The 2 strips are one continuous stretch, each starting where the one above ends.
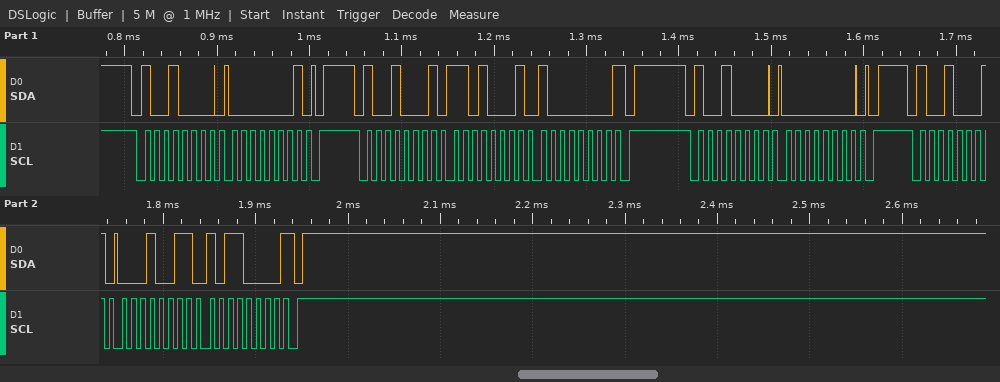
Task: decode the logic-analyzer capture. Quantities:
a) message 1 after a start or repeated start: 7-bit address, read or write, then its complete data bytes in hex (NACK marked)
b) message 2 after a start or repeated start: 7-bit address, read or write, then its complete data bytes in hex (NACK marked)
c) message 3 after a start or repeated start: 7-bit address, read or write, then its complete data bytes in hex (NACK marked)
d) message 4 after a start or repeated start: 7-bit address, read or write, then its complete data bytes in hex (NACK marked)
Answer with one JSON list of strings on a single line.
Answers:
["0x48 write: 01", "0x48 read: D1 80 NACK", "0x48 write: 00", "0x48 read: 13 B0 NACK"]
